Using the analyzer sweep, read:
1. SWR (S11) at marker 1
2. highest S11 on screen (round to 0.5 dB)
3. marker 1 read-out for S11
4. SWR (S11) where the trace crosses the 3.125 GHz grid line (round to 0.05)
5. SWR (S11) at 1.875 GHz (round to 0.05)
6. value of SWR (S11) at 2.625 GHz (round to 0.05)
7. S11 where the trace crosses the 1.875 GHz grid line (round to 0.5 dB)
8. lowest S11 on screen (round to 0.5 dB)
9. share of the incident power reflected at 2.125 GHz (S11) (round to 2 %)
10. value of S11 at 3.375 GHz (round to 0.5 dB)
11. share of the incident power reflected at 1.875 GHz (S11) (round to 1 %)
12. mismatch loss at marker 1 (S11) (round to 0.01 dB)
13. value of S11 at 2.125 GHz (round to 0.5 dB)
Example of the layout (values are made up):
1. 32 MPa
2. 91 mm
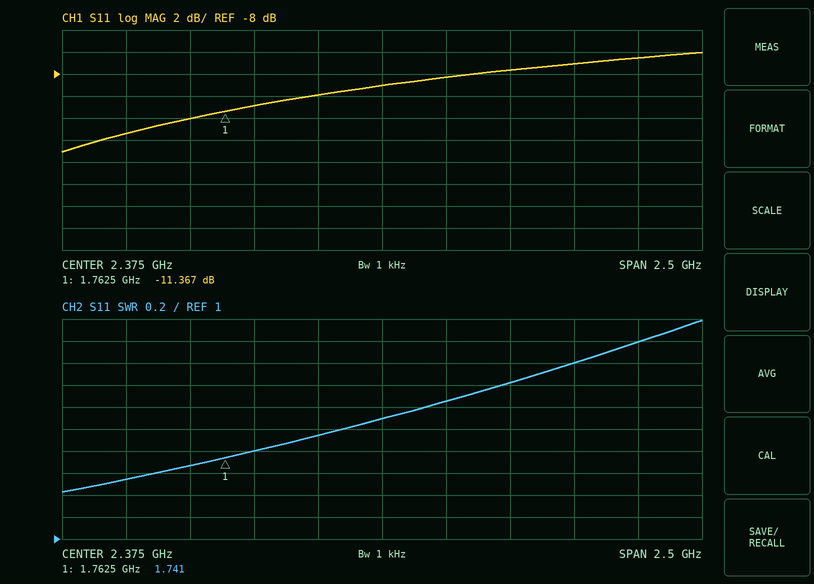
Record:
1. 1.741
2. -6.0 dB
3. -11.367 dB
4. 2.60
5. 1.80
6. 2.25
7. -11.0 dB
8. -15.0 dB
9. 10 %
10. -6.5 dB
11. 8 %
12. 0.33 dB
13. -10.0 dB
